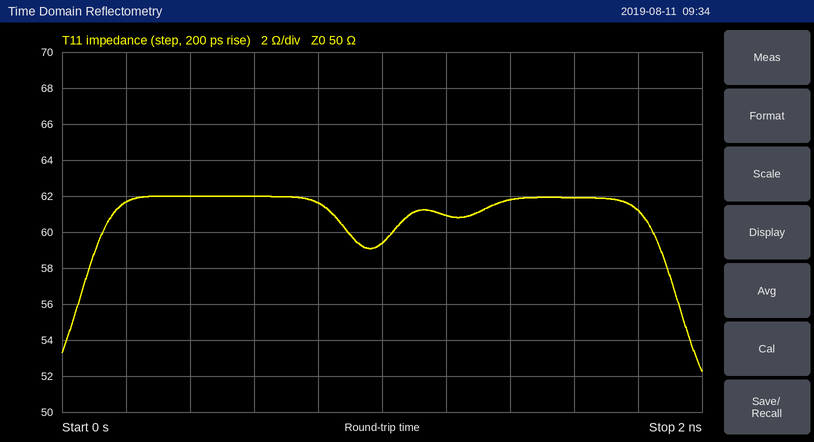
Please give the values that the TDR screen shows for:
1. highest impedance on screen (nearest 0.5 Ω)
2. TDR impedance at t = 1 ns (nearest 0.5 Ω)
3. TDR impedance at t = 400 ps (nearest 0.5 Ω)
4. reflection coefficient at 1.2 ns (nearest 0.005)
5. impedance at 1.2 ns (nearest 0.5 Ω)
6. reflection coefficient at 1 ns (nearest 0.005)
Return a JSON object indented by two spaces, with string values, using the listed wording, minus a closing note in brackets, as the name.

{
  "highest impedance on screen": "62.0 Ω",
  "TDR impedance at t = 1 ns": "59.5 Ω",
  "TDR impedance at t = 400 ps": "62.0 Ω",
  "reflection coefficient at 1.2 ns": "+0.100",
  "impedance at 1.2 ns": "61.0 Ω",
  "reflection coefficient at 1 ns": "+0.085"
}
